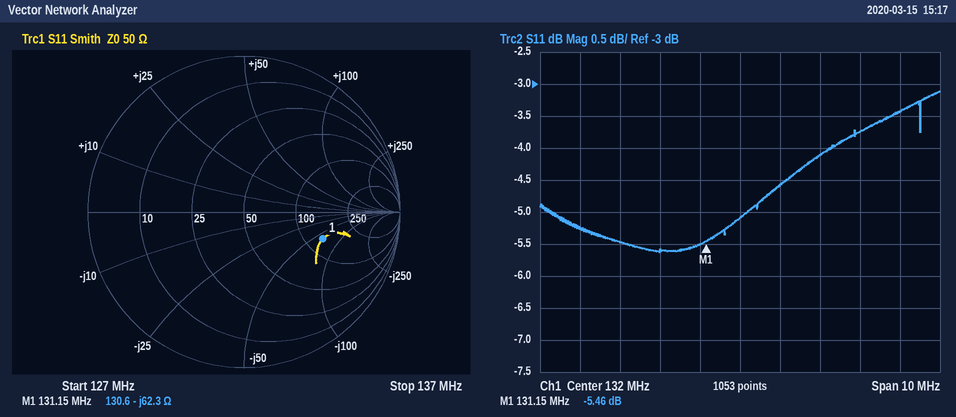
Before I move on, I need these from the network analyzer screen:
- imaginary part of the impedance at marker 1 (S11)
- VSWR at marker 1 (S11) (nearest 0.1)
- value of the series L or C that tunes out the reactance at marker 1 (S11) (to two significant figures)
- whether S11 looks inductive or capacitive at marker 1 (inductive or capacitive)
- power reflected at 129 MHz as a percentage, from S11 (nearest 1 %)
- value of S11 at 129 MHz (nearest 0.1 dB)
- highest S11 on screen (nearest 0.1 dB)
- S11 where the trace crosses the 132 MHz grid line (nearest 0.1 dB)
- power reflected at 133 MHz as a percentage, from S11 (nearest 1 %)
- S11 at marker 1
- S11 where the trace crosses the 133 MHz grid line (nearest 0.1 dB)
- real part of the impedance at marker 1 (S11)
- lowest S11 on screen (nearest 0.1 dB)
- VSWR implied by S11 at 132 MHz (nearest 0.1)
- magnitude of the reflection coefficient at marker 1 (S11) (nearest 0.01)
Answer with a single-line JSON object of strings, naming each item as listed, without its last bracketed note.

{"imaginary part of the impedance at marker 1": "-62.3 Ω", "VSWR at marker 1 (S11)": "3.3", "value of the series L or C that tunes out the reactance at marker 1 (S11)": "76 nH", "whether S11 looks inductive or capacitive at marker 1": "capacitive", "power reflected at 129 MHz as a percentage, from S11": "28 %", "value of S11 at 129 MHz": "-5.5 dB", "highest S11 on screen": "-3.1 dB", "S11 where the trace crosses the 132 MHz grid line": "-5.1 dB", "power reflected at 133 MHz as a percentage, from S11": "35 %", "S11 at marker 1": "-5.46 dB", "S11 where the trace crosses the 133 MHz grid line": "-4.6 dB", "real part of the impedance at marker 1": "130.6 Ω", "lowest S11 on screen": "-5.6 dB", "VSWR implied by S11 at 132 MHz": "3.5", "magnitude of the reflection coefficient at marker 1 (S11)": "0.53"}
